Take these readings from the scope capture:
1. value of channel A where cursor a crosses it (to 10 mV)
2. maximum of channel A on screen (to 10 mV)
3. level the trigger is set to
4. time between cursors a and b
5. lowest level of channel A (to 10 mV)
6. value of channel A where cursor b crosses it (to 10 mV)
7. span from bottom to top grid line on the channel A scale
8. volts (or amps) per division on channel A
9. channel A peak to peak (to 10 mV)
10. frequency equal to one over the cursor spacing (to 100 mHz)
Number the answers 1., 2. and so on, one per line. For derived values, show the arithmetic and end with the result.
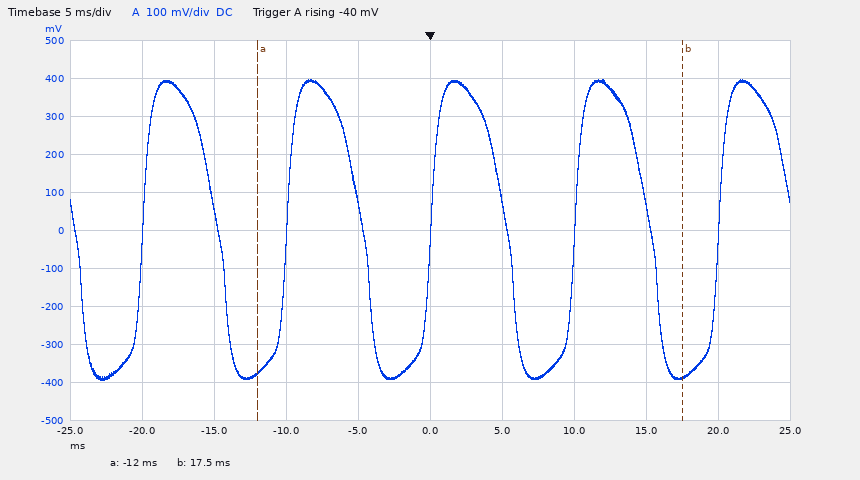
1. -370 mV
2. 400 mV
3. -40 mV
4. 17.5 ms − (-12 ms) = 29.5 ms
5. -390 mV
6. -390 mV
7. 1 V
8. 100 mV
9. 400 mV − (-390 mV) = 790 mV
10. 1 / 29.5 ms ≈ 33.9 Hz
